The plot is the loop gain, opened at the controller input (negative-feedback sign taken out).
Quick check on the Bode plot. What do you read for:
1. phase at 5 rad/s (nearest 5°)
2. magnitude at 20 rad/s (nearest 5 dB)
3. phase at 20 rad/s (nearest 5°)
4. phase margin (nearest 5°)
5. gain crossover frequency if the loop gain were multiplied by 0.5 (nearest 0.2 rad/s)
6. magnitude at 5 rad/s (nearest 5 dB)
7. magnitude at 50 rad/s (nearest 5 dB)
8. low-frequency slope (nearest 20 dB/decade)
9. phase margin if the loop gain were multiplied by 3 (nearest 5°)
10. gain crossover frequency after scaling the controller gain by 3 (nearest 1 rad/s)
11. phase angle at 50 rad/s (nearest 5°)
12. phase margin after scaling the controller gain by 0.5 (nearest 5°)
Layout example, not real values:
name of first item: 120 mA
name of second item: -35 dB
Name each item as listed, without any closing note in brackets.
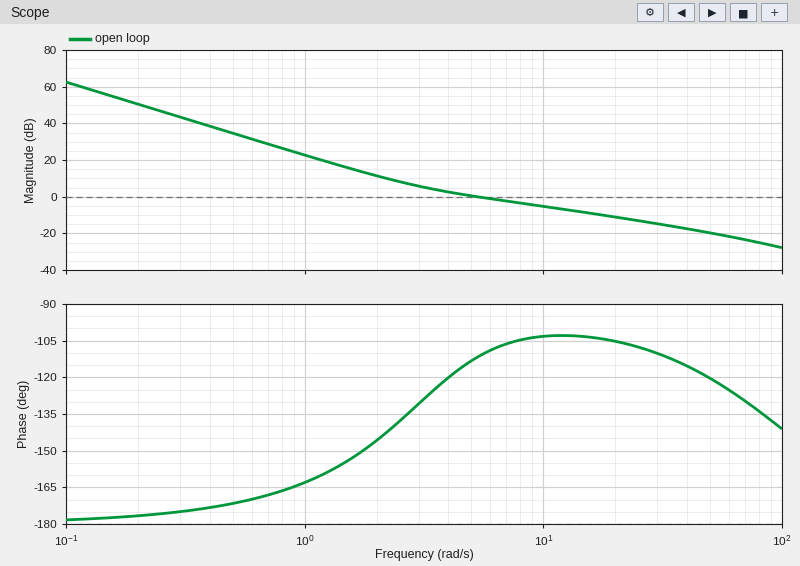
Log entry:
phase at 5 rad/s: -115°
magnitude at 20 rad/s: -10 dB
phase at 20 rad/s: -105°
phase margin: 70°
gain crossover frequency if the loop gain were multiplied by 0.5: 3.0 rad/s
magnitude at 5 rad/s: 0 dB
magnitude at 50 rad/s: -20 dB
low-frequency slope: -40 dB/decade
phase margin if the loop gain were multiplied by 3: 75°
gain crossover frequency after scaling the controller gain by 3: 17 rad/s
phase angle at 50 rad/s: -120°
phase margin after scaling the controller gain by 0.5: 50°
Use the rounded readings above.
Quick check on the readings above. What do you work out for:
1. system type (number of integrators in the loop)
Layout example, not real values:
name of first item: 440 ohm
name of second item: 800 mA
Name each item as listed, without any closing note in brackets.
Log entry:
system type: 2
